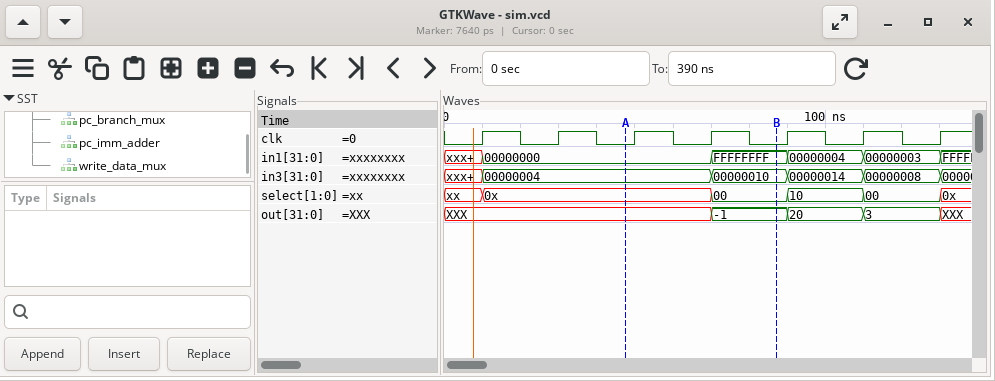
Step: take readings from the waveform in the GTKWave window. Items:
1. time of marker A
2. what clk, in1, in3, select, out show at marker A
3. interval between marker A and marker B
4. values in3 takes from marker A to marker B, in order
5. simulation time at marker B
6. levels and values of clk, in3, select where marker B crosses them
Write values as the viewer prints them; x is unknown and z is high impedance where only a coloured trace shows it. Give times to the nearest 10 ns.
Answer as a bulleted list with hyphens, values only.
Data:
- 50 ns
- clk=0, in1=00000000, in3=00000004, select=0x, out=XXX
- 40 ns
- 00000004, 00000010
- 90 ns
- clk=0, in3=00000010, select=00
